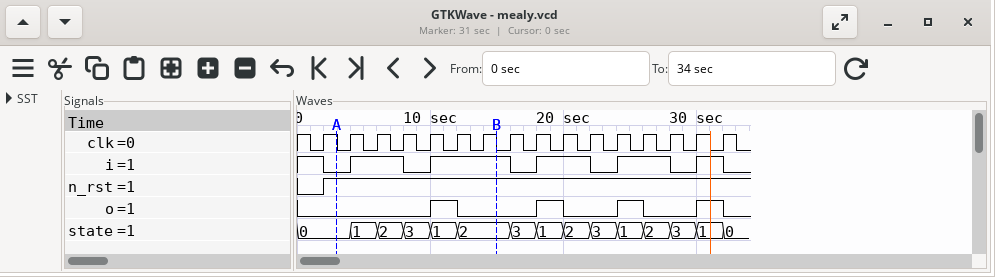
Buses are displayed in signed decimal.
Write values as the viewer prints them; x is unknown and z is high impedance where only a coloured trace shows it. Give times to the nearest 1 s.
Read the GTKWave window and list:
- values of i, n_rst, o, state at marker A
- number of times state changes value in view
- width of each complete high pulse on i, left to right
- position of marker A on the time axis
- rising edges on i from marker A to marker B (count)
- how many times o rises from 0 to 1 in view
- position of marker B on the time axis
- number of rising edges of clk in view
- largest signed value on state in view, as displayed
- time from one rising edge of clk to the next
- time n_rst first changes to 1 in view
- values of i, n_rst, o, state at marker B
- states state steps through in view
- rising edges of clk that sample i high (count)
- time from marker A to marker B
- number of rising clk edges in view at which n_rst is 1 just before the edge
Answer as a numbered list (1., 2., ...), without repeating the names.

1. i=0, n_rst=1, o=0, state=0
2. 14
3. 4 s, 6 s, 4 s, 4 s, 2 s
4. 3 s
5. 2
6. 4
7. 15 s
8. 16
9. 3
10. 2 s
11. 2 s
12. i=1, n_rst=1, o=0, state=2
13. 0, 1, 2, 3, 1, 2, 3, 1, 2, 3, 1, 2, 3, 1, 0
14. 11
15. 12 s
16. 15
